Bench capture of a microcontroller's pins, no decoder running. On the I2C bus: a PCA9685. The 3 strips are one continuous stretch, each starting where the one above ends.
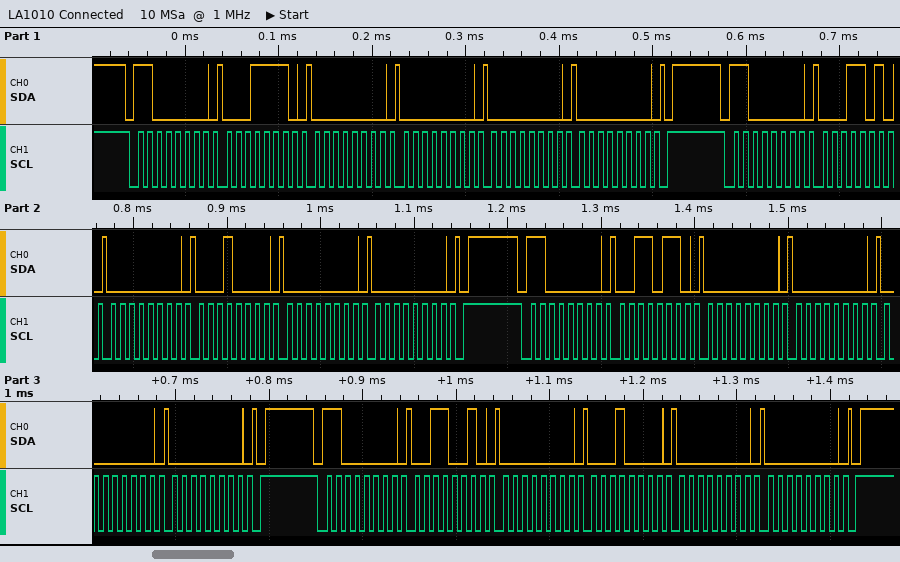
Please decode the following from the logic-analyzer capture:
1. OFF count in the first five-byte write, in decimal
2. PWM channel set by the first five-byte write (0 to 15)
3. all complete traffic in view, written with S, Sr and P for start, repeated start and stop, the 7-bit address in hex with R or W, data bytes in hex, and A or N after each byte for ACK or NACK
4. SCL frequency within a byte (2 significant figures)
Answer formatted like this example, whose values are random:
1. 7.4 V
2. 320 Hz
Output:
1. 0
2. 6
3. S 60W A 1E A 00 A 00 A 00 A 00 A P S 60W A 1A A 00 A 10 A 00 A 00 A P S 60W A 36 A 00 A 00 A 00 A 00 A P S 60W A 32 A 00 A 10 A 00 A 00 A P
4. 100 kHz
